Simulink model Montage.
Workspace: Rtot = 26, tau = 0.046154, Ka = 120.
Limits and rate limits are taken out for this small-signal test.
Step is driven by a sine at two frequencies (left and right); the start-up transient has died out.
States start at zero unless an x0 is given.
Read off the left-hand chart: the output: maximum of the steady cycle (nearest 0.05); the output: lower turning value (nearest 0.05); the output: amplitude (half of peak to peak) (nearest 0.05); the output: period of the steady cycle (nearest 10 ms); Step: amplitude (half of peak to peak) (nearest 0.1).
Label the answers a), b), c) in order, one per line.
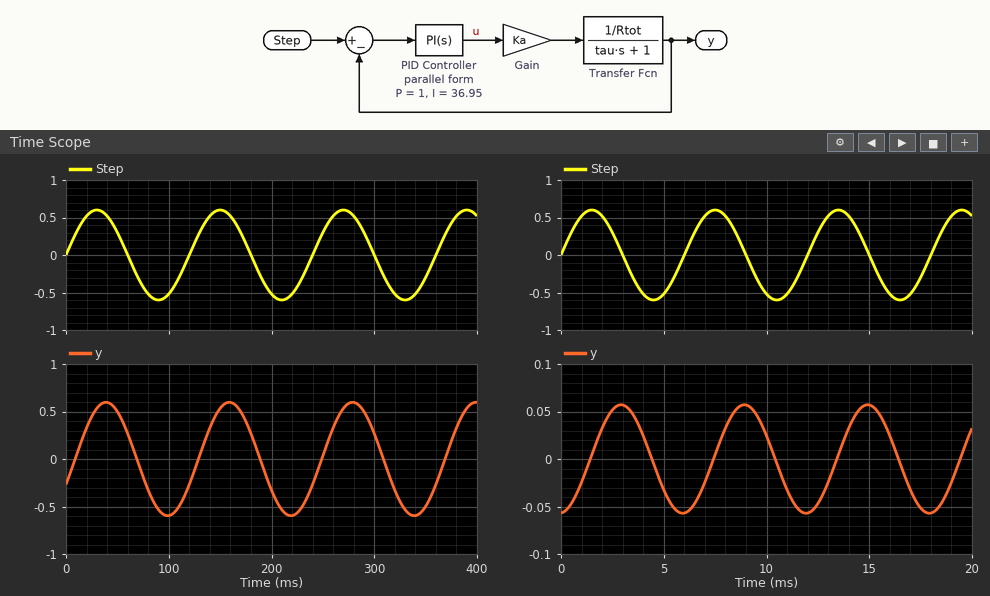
a) 0.60
b) -0.60
c) 0.60
d) 120 ms
e) 0.6
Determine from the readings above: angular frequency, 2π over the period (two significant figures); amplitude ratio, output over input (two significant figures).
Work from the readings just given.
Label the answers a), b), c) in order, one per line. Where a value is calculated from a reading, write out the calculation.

a) 2π / 120 = 0.052 rad/ms
b) 0.6 / 0.6 = 1.0
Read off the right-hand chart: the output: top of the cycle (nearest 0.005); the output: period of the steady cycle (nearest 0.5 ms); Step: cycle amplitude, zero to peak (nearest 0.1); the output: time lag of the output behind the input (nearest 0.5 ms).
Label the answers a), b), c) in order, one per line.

a) 0.055
b) 6.0 ms
c) 0.6
d) 1.5 ms
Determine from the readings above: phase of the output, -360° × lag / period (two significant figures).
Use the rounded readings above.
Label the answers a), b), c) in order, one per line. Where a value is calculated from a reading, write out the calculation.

a) -360 × 1.5 / 6 = -90°
